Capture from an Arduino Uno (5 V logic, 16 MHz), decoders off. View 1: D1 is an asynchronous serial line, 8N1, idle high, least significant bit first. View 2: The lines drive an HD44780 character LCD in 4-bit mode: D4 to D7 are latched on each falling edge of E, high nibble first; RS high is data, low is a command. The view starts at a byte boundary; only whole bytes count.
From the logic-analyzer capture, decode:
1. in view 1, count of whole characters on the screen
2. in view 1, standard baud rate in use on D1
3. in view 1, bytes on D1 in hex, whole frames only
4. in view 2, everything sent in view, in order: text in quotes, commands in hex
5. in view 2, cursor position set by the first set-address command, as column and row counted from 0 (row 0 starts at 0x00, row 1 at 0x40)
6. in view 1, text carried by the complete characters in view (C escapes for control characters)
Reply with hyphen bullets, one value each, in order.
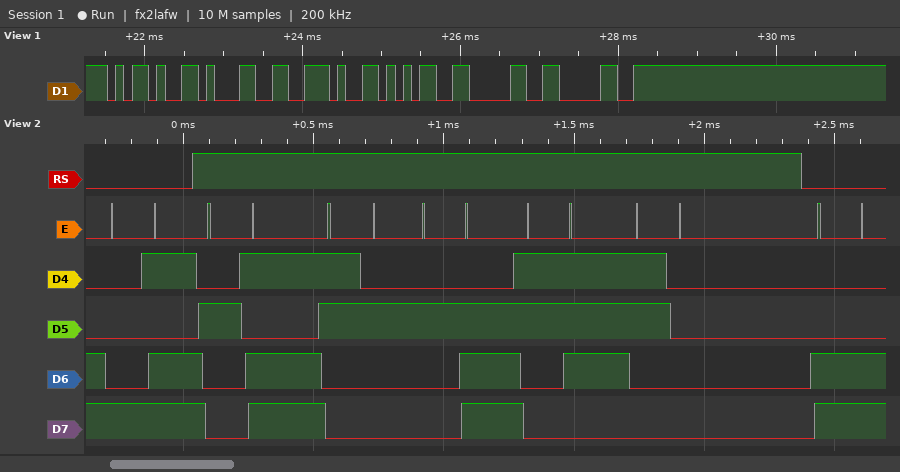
- 6
- 9600 baud
- 2D 31 2E 35 30 30
- 0x8D "-2.70" 0xCC
- column 13, row 0
- "-1.500"
